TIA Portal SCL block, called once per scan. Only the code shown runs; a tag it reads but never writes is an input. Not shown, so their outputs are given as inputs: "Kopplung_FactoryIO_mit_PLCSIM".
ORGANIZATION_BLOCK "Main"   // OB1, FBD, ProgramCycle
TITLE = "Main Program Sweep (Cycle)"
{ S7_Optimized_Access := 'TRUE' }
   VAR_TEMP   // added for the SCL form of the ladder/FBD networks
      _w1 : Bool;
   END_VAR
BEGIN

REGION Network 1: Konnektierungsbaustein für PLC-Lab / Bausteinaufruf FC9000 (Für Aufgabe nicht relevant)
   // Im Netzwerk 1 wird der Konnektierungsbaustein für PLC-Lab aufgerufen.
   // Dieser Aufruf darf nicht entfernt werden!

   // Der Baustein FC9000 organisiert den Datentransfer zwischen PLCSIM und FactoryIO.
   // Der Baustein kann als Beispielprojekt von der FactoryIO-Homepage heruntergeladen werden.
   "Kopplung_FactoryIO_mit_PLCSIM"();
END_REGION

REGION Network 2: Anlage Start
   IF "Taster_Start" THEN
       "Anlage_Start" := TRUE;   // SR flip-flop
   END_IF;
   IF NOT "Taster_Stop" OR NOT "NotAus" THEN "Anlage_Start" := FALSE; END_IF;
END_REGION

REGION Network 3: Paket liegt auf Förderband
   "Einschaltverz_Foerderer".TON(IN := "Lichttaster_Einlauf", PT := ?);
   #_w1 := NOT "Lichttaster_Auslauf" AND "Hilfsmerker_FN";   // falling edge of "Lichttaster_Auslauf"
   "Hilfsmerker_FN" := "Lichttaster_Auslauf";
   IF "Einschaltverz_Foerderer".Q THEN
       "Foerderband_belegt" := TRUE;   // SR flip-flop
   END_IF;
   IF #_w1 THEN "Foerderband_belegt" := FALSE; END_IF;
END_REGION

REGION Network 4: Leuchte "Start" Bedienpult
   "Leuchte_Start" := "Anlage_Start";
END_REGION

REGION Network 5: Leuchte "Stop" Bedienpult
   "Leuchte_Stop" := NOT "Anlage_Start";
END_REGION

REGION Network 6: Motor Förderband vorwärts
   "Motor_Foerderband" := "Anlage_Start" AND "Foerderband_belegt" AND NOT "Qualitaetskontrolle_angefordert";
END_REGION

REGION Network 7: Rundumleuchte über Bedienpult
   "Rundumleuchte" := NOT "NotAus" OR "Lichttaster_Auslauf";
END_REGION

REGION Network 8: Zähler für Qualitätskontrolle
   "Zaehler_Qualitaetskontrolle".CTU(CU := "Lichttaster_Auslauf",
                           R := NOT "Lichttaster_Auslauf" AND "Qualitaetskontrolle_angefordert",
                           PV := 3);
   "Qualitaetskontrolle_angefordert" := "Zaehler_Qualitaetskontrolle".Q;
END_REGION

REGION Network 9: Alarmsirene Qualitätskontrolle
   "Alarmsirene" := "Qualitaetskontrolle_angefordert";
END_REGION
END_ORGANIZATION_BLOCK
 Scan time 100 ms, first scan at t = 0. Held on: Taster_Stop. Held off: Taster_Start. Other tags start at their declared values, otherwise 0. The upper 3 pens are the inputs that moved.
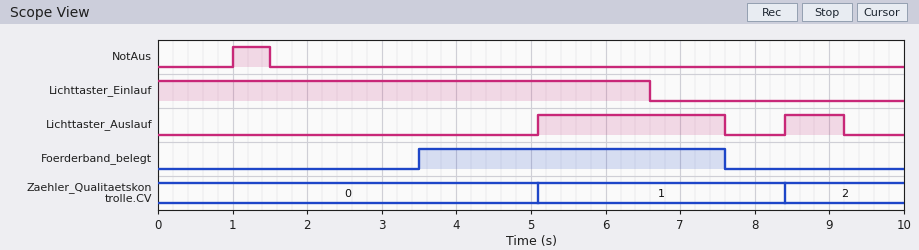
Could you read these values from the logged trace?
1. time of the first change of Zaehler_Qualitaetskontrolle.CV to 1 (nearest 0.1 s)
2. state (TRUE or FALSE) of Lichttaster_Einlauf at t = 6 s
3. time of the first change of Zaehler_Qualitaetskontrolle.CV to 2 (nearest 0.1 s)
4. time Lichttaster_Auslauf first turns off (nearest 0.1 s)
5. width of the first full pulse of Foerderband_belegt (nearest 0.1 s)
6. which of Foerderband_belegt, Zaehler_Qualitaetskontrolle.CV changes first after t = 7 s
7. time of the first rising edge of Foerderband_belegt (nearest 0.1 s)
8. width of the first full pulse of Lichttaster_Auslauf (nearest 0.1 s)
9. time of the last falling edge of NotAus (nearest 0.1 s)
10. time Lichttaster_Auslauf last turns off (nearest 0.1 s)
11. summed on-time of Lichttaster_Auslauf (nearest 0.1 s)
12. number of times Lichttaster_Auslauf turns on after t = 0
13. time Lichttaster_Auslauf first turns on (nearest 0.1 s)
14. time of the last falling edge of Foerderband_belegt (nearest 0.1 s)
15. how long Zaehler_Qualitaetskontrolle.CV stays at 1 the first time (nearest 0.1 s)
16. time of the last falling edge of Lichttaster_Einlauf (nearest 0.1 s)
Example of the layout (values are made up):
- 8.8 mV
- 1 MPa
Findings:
- 5.1 s
- TRUE
- 8.4 s
- 7.6 s
- 4.1 s
- Foerderband_belegt
- 3.5 s
- 2.5 s
- 1.5 s
- 9.2 s
- 3.3 s
- 2
- 5.1 s
- 7.6 s
- 3.3 s
- 6.6 s
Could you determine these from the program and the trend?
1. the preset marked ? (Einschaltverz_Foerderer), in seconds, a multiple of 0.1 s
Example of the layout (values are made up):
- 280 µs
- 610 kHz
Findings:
- 3.5 s
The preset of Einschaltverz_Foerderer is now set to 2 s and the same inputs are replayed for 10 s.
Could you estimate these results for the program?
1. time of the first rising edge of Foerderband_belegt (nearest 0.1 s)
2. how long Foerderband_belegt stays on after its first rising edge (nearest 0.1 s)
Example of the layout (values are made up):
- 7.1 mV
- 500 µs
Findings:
- 2.0 s
- 5.6 s
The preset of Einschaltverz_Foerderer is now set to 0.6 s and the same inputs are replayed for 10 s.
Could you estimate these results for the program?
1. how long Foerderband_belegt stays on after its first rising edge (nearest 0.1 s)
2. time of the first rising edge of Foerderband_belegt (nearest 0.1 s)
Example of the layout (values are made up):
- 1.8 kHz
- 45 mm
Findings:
- 7.0 s
- 0.6 s
